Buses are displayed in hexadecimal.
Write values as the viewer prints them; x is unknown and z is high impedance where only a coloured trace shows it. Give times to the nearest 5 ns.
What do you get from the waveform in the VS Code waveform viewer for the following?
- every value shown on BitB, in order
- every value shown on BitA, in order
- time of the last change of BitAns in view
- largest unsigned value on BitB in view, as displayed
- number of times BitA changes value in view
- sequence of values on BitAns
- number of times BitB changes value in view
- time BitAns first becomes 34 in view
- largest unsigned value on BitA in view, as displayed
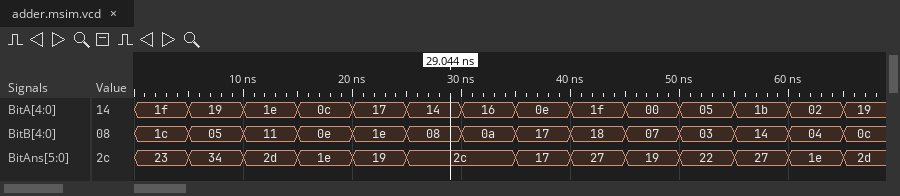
1c, 05, 11, 0e, 1e, 08, 0a, 17, 18, 07, 03, 14, 04, 0c
1f, 19, 1e, 0c, 17, 14, 16, 0e, 1f, 00, 05, 1b, 02, 19
65 ns
1e
13
23, 34, 2d, 1e, 19, 2c, 17, 27, 19, 22, 27, 1e, 2d
13
5 ns
1f
